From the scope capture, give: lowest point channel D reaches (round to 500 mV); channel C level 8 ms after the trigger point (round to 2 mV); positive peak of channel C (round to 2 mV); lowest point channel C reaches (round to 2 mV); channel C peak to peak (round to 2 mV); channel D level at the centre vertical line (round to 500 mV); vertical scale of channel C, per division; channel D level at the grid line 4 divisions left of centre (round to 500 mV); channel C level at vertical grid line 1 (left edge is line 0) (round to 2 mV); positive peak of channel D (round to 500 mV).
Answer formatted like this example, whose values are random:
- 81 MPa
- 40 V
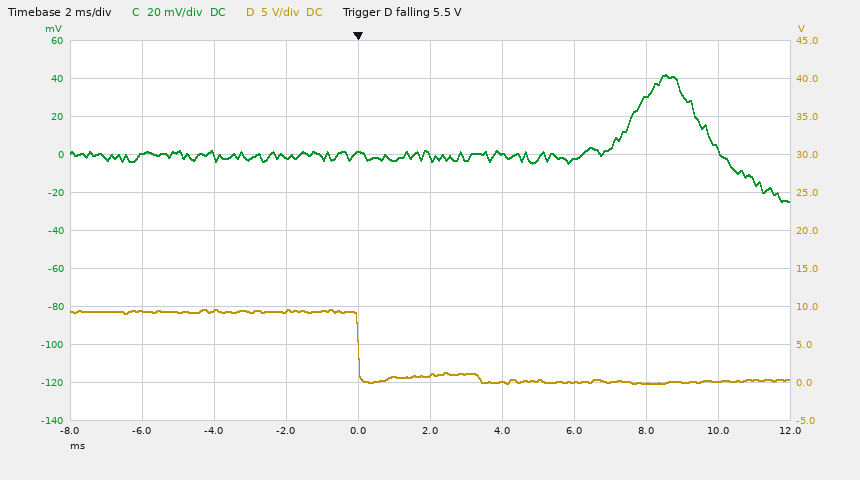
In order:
- 0.0 V
- 30 mV
- 42 mV
- -24 mV
- 66 mV
- 1.0 V
- 20 mV
- 9.5 V
- 0 mV
- 9.5 V
